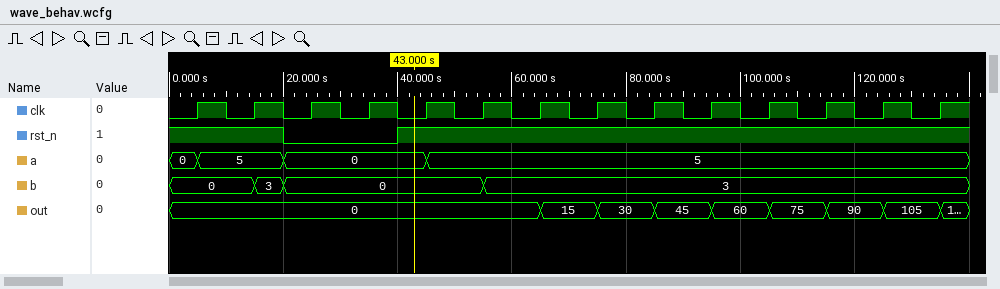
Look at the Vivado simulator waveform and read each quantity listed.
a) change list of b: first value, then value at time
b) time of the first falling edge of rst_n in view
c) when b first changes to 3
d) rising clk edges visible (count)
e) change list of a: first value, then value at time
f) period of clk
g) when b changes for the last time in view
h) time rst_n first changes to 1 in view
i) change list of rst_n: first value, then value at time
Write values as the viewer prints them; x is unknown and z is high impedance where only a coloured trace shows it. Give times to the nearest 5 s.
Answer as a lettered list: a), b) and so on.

a) 0, 3 at 15 s, 0 at 20 s, 3 at 55 s
b) 20 s
c) 15 s
d) 14
e) 0, 5 at 5 s, 0 at 20 s, 5 at 45 s
f) 10 s
g) 55 s
h) 40 s
i) 1, 0 at 20 s, 1 at 40 s
